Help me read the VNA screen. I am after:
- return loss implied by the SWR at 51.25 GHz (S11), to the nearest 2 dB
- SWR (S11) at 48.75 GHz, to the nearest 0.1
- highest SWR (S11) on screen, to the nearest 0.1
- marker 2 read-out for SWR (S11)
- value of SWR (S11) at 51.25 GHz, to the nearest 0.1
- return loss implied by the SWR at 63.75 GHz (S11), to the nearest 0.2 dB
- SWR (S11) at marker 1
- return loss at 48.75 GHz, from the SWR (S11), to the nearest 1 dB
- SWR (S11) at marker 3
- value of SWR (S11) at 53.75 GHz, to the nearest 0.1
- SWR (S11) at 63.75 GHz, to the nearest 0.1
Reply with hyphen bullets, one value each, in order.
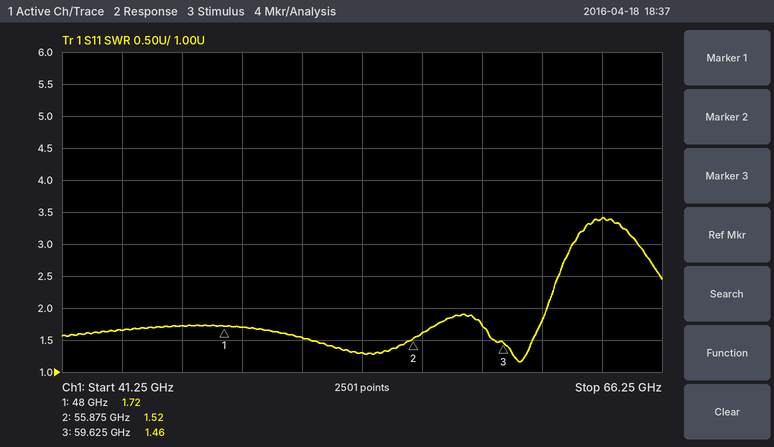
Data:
- 14 dB
- 1.7
- 3.4
- 1.52
- 1.5
- 5.2 dB
- 1.72
- 12 dB
- 1.46
- 1.3
- 3.4
